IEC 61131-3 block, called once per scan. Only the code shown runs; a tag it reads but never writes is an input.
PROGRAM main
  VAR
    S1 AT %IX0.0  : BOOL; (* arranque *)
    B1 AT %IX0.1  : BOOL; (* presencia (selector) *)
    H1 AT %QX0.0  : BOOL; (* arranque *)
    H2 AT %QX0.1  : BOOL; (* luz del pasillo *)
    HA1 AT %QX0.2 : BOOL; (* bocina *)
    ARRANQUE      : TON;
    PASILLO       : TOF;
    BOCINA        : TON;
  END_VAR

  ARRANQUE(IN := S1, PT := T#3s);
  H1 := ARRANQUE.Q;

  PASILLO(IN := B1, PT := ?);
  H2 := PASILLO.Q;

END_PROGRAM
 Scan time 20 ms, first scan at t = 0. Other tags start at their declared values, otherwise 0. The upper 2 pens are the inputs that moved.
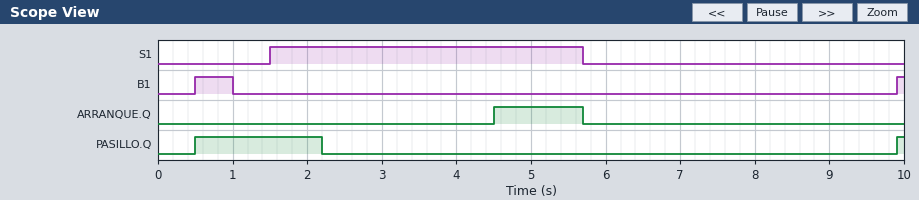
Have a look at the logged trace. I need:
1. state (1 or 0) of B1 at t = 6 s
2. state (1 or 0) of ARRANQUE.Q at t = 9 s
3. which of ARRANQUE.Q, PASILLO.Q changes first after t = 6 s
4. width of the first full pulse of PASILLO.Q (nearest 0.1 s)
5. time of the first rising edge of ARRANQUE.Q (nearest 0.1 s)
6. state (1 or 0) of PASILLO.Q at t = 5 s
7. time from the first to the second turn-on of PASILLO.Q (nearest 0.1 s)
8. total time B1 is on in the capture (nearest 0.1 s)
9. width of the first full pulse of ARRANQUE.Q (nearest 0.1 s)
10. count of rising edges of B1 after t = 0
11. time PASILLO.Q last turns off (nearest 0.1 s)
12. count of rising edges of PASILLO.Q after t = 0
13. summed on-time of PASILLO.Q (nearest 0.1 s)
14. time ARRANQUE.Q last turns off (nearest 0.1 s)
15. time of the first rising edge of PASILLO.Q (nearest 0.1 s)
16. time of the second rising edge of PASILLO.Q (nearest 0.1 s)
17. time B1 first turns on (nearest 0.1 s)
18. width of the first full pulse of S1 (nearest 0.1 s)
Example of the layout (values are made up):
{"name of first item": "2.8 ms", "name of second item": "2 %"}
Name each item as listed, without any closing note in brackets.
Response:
{"state (1 or 0) of B1 at t = 6 s": "0", "state (1 or 0) of ARRANQUE.Q at t = 9 s": "0", "which of ARRANQUE.Q, PASILLO.Q changes first after t = 6 s": "PASILLO.Q", "width of the first full pulse of PASILLO.Q": "1.7 s", "time of the first rising edge of ARRANQUE.Q": "4.5 s", "state (1 or 0) of PASILLO.Q at t = 5 s": "0", "time from the first to the second turn-on of PASILLO.Q": "9.4 s", "total time B1 is on in the capture": "0.6 s", "width of the first full pulse of ARRANQUE.Q": "1.2 s", "count of rising edges of B1 after t = 0": "2", "time PASILLO.Q last turns off": "2.2 s", "count of rising edges of PASILLO.Q after t = 0": "2", "summed on-time of PASILLO.Q": "1.8 s", "time ARRANQUE.Q last turns off": "5.7 s", "time of the first rising edge of PASILLO.Q": "0.5 s", "time of the second rising edge of PASILLO.Q": "9.9 s", "time B1 first turns on": "0.5 s", "width of the first full pulse of S1": "4.2 s"}
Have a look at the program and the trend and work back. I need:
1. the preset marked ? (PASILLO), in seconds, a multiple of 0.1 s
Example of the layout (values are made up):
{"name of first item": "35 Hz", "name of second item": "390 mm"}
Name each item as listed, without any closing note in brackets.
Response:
{"the preset marked ? (PASILLO), in seconds, a multiple of 0.1 s": "1.2 s"}
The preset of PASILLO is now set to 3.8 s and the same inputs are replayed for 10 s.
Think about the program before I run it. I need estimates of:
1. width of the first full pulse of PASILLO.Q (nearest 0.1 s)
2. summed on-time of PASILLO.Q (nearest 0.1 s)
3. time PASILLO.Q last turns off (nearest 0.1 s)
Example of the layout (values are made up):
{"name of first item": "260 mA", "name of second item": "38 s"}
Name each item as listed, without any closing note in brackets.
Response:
{"width of the first full pulse of PASILLO.Q": "4.3 s", "summed on-time of PASILLO.Q": "4.4 s", "time PASILLO.Q last turns off": "4.8 s"}
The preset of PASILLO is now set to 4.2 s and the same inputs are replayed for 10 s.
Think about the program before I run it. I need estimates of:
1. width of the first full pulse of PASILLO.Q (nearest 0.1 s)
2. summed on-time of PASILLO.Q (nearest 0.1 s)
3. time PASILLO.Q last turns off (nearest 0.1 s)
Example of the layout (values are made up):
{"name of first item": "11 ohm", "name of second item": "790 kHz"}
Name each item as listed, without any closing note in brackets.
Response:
{"width of the first full pulse of PASILLO.Q": "4.7 s", "summed on-time of PASILLO.Q": "4.8 s", "time PASILLO.Q last turns off": "5.2 s"}
